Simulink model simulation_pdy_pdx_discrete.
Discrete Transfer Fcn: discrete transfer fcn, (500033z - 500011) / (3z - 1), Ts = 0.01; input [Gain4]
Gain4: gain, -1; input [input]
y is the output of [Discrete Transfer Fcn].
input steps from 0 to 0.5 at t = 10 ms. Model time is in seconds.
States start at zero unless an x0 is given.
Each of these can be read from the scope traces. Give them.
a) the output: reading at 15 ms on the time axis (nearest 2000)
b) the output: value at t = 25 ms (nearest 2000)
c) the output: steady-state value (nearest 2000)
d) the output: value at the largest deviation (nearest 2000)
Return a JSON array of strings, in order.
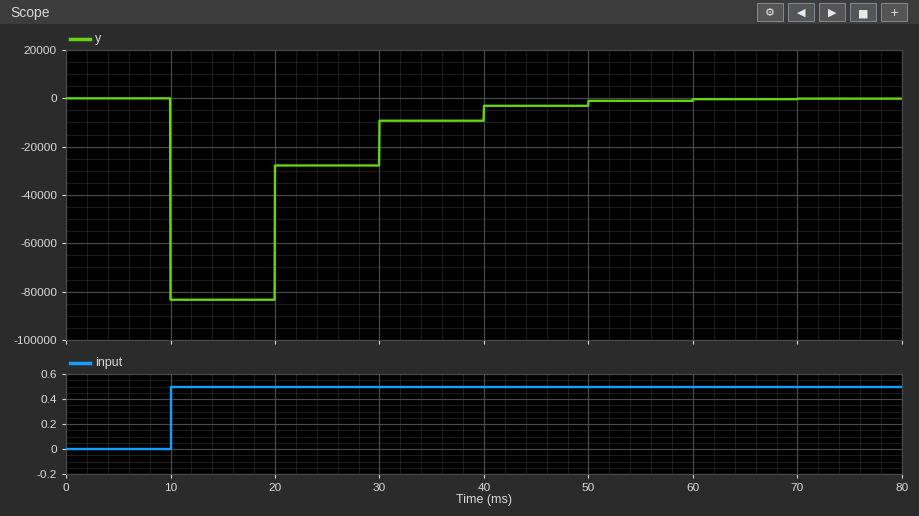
["-84000", "-28000", "0", "-84000"]
